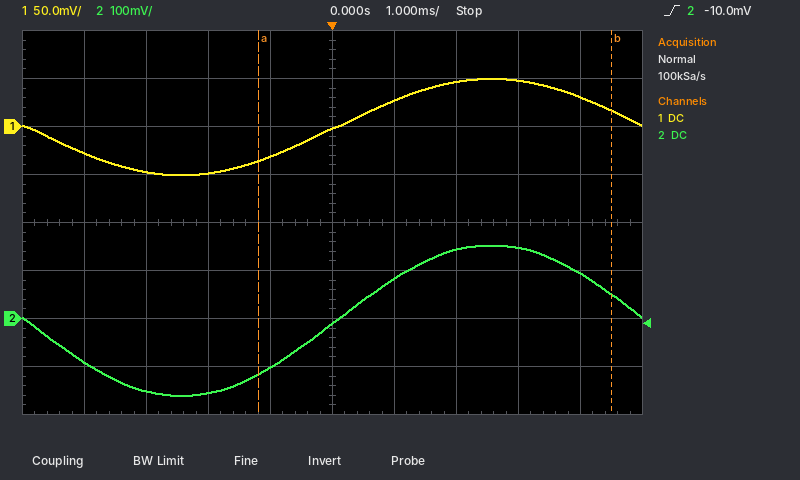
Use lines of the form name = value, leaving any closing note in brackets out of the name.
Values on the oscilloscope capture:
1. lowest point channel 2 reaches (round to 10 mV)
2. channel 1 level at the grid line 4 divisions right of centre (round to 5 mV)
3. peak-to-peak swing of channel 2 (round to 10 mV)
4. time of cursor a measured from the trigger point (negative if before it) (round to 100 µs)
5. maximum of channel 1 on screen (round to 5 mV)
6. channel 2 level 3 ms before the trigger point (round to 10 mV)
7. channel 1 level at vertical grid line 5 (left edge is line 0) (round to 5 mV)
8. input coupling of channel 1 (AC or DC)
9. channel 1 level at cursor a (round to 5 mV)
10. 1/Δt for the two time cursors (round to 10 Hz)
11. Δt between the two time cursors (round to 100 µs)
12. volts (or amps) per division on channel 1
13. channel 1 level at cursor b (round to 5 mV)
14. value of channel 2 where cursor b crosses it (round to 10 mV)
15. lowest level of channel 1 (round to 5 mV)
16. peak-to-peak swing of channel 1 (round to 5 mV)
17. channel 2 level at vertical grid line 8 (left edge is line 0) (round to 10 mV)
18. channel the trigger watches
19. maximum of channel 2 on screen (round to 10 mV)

lowest point channel 2 reaches = -160 mV
channel 1 level at the grid line 4 divisions right of centre = 30 mV
peak-to-peak swing of channel 2 = 310 mV
time of cursor a measured from the trigger point (negative if before it) = -1.2 ms
maximum of channel 1 on screen = 50 mV
channel 2 level 3 ms before the trigger point = -150 mV
channel 1 level at vertical grid line 5 (left edge is line 0) = 0 mV
input coupling of channel 1 = DC
channel 1 level at cursor a = -35 mV
1/Δt for the two time cursors = 180 Hz
Δt between the two time cursors = 5.7 ms
volts (or amps) per division on channel 1 = 50 mV
channel 1 level at cursor b = 15 mV
value of channel 2 where cursor b crosses it = 50 mV
lowest level of channel 1 = -50 mV
peak-to-peak swing of channel 1 = 100 mV
channel 2 level at vertical grid line 8 (left edge is line 0) = 150 mV
channel the trigger watches = channel 2
maximum of channel 2 on screen = 150 mV
